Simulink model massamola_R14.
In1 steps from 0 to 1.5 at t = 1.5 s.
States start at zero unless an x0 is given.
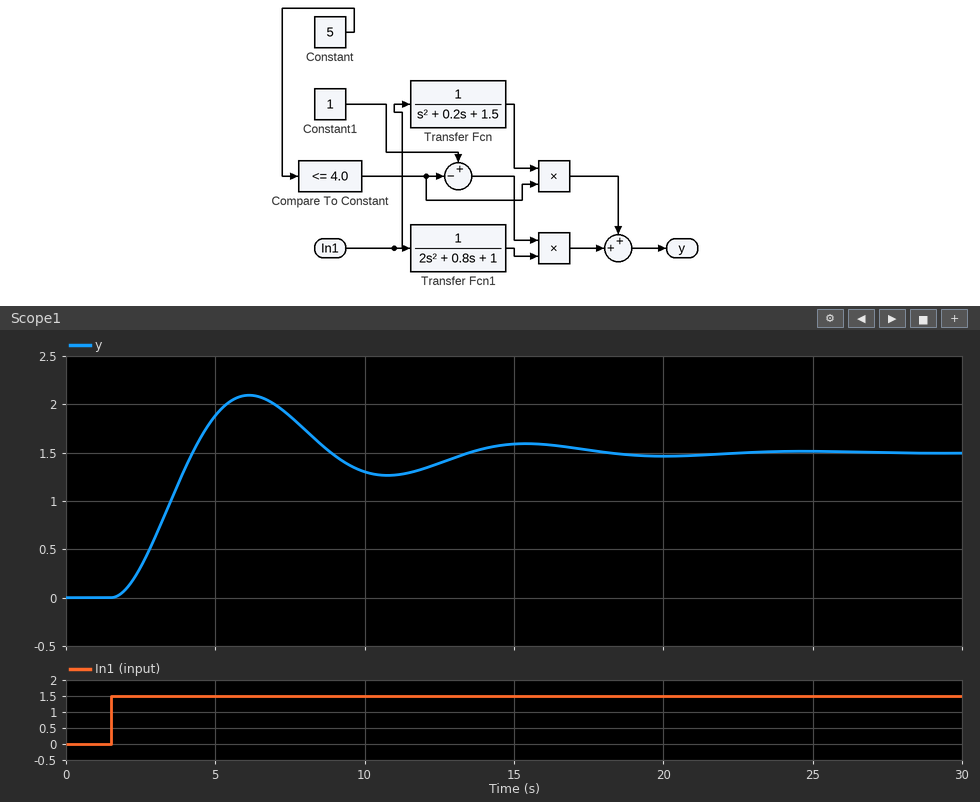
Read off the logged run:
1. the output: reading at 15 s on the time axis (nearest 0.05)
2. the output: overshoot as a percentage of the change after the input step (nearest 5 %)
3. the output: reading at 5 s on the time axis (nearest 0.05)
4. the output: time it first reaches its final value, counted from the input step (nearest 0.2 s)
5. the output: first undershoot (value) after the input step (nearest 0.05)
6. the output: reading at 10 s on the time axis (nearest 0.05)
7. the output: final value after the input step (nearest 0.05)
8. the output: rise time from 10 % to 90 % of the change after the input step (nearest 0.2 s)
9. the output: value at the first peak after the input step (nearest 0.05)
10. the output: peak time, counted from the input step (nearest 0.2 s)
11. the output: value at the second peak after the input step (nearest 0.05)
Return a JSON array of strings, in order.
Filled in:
["1.60", "40 %", "1.90", "2.8 s", "1.25", "1.30", "1.50", "1.8 s", "2.10", "4.6 s", "1.60"]
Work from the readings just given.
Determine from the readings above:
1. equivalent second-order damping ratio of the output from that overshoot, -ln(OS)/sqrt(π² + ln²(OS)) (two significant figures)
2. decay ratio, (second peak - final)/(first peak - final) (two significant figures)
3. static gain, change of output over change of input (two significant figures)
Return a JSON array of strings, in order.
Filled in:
["0.28", "0.17", "1.0"]
